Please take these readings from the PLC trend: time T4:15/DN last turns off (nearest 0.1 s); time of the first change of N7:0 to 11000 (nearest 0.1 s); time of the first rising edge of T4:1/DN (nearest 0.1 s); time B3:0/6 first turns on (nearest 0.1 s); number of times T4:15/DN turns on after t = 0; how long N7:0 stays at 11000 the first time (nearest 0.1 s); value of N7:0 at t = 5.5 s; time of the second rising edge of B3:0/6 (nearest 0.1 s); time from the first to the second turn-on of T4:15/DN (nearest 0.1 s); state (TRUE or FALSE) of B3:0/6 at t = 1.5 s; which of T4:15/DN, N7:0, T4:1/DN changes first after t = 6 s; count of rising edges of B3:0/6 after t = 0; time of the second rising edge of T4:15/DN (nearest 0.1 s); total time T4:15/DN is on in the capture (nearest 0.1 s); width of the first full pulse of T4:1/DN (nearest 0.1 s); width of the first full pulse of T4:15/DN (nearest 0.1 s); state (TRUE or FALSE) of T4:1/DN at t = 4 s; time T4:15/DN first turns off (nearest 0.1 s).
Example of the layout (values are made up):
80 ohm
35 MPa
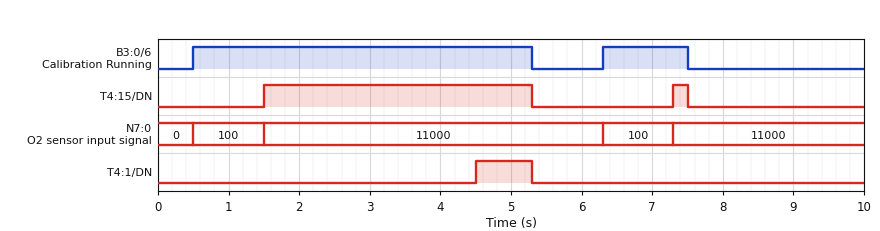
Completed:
7.5 s
1.5 s
4.5 s
0.5 s
2
4.8 s
11000
6.3 s
5.8 s
TRUE
N7:0
2
7.3 s
4.0 s
0.8 s
3.8 s
FALSE
5.3 s
